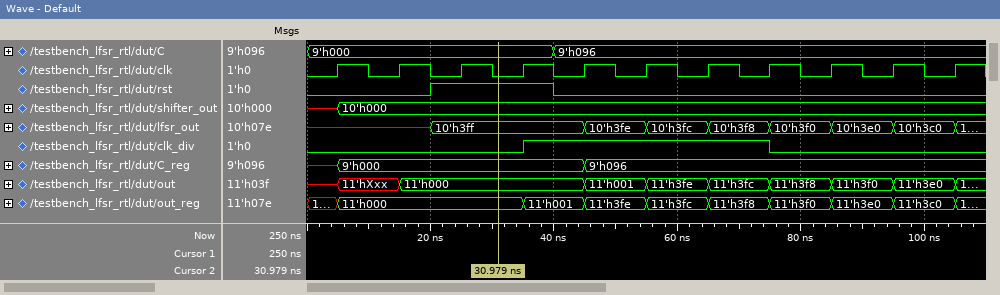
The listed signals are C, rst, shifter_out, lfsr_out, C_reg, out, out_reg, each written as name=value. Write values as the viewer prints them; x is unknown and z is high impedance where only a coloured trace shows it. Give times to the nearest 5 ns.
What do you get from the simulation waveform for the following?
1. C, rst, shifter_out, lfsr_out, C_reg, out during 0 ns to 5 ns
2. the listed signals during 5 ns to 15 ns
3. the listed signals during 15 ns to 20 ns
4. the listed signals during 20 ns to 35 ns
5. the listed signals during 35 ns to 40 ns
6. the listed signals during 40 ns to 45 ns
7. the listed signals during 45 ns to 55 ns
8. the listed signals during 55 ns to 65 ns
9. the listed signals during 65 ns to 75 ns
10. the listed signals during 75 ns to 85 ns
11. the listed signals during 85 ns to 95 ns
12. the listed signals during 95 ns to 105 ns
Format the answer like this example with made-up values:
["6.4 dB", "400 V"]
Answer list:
["C=9'h000, rst=0, shifter_out=x, lfsr_out=x, C_reg=x, out=x", "C=9'h000, rst=0, shifter_out=10'h000, lfsr_out=x, C_reg=9'h000, out=11'hXxx, out_reg=11'h000", "C=9'h000, rst=0, shifter_out=10'h000, lfsr_out=x, C_reg=9'h000, out=11'h000, out_reg=11'h000", "C=9'h000, rst=1, shifter_out=10'h000, lfsr_out=10'h3ff, C_reg=9'h000, out=11'h000, out_reg=11'h000", "C=9'h000, rst=1, shifter_out=10'h000, lfsr_out=10'h3ff, C_reg=9'h000, out=11'h000, out_reg=11'h001", "C=9'h096, rst=0, shifter_out=10'h000, lfsr_out=10'h3ff, C_reg=9'h000, out=11'h000, out_reg=11'h001", "C=9'h096, rst=0, shifter_out=10'h000, lfsr_out=10'h3fe, C_reg=9'h096, out=11'h001, out_reg=11'h3fe", "C=9'h096, rst=0, shifter_out=10'h000, lfsr_out=10'h3fc, C_reg=9'h096, out=11'h3fe, out_reg=11'h3fc", "C=9'h096, rst=0, shifter_out=10'h000, lfsr_out=10'h3f8, C_reg=9'h096, out=11'h3fc, out_reg=11'h3f8", "C=9'h096, rst=0, shifter_out=10'h000, lfsr_out=10'h3f0, C_reg=9'h096, out=11'h3f8, out_reg=11'h3f0", "C=9'h096, rst=0, shifter_out=10'h000, lfsr_out=10'h3e0, C_reg=9'h096, out=11'h3f0, out_reg=11'h3e0", "C=9'h096, rst=0, shifter_out=10'h000, lfsr_out=10'h3c0, C_reg=9'h096, out=11'h3e0, out_reg=11'h3c0"]
